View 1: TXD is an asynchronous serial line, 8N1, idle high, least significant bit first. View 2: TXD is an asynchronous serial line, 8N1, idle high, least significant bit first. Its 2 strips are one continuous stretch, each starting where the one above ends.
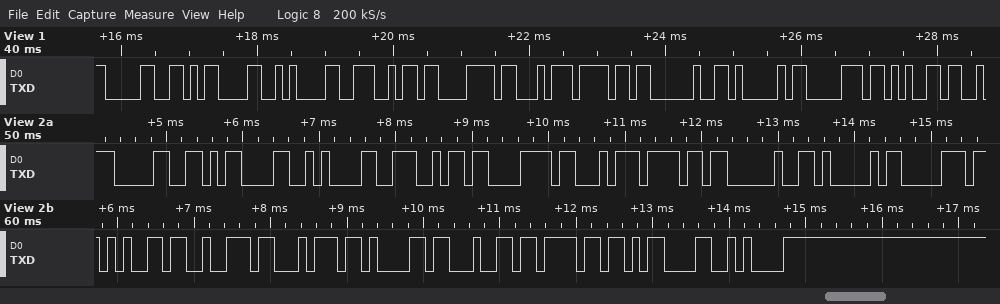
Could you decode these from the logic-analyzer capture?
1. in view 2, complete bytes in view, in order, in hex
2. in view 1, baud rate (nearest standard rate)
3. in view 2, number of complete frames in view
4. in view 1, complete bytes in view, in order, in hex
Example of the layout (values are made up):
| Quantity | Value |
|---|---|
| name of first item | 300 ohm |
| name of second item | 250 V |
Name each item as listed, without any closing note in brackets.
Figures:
| Quantity | Value |
|---|---|
| in view 2, complete bytes in view, in order, in hex | 30 0D 0A 4E C3 A3 6F 20 41 70 65 72 74 61 64 6F 0D 0A |
| in view 1, baud rate | 9600 baud |
| in view 2, number of complete frames in view | 18 |
| in view 1, complete bytes in view, in order, in hex | 30 0D 0A 4E C3 A3 6F 20 41 70 65 |
